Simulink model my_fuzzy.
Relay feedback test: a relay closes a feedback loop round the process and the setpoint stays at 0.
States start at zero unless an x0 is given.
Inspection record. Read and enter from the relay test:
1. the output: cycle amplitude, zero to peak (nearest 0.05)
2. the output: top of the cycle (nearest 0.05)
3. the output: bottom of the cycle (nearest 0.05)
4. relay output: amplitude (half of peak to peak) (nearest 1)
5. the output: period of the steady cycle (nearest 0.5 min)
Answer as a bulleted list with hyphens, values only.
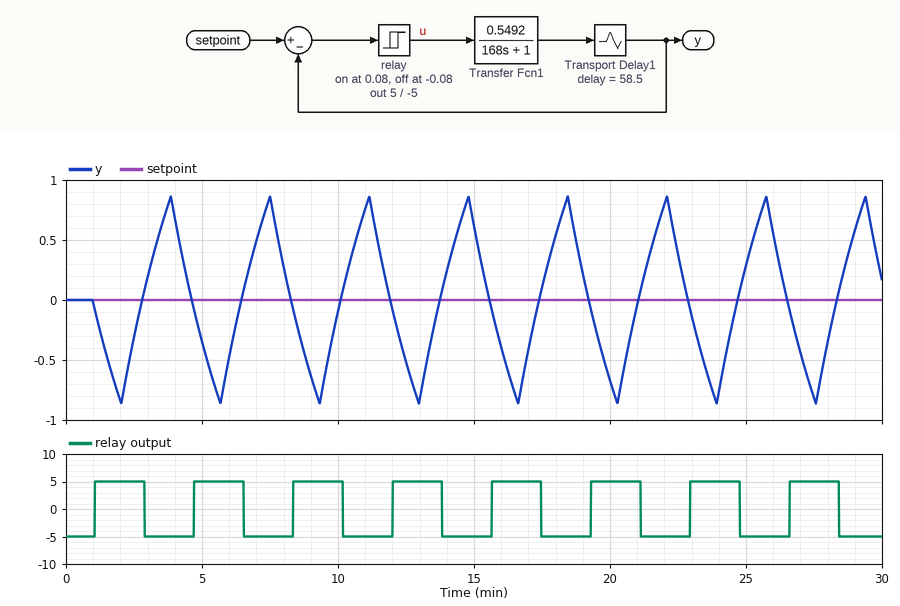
- 0.85
- 0.85
- -0.85
- 5
- 3.5 min
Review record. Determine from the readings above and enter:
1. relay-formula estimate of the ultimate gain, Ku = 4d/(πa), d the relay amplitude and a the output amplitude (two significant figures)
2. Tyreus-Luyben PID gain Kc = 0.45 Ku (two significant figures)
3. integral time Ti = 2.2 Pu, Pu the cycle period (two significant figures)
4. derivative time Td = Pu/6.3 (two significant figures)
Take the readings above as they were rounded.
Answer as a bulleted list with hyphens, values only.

- 7.5
- 3.4
- 7.7 min
- 0.56 min
